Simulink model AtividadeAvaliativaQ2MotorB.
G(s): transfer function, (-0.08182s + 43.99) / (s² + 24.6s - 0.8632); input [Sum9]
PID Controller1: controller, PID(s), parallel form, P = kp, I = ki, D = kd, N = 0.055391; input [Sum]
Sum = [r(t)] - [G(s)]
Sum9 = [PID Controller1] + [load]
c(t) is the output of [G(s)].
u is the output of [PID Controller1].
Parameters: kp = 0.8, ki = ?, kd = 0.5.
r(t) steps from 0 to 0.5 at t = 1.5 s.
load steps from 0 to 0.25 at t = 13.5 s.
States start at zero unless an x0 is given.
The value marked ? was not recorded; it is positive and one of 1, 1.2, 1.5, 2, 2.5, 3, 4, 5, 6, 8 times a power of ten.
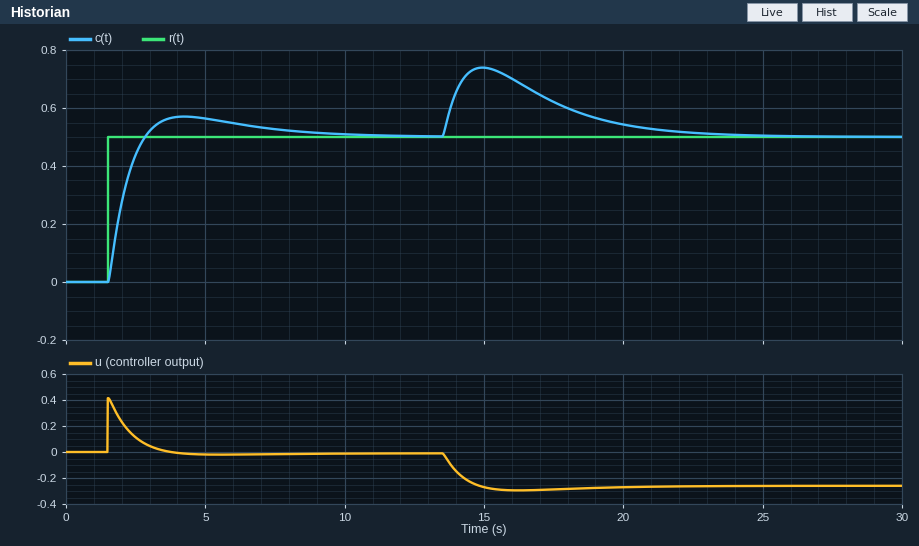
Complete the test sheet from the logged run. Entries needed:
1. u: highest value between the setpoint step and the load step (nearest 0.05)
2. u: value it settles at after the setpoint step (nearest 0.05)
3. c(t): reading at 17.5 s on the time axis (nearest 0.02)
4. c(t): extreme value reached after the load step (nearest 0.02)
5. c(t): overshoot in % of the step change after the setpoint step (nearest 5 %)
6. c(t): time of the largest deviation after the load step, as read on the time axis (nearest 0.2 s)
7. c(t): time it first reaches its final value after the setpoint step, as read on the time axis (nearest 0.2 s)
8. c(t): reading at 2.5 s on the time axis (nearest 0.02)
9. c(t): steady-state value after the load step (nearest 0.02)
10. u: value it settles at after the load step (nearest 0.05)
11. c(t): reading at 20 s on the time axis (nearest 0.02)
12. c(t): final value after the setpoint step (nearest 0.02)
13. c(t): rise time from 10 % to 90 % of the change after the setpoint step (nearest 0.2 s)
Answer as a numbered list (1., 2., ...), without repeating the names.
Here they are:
1. 0.40
2. 0.00
3. 0.62
4. 0.74
5. 15 %
6. 15.0 s
7. 2.8 s
8. 0.44
9. 0.50
10. -0.25
11. 0.54
12. 0.50
13. 1.0 s
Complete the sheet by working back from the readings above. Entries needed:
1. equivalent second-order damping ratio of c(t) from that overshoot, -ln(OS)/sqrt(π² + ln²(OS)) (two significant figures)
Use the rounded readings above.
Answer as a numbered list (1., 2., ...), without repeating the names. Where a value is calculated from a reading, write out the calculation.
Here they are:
1. ln(0.15) = -1.897; 1.897 / sqrt(9.870 + 3.599) = 0.52
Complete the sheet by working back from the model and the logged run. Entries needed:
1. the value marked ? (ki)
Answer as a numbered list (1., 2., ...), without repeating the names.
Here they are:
1. 0.25
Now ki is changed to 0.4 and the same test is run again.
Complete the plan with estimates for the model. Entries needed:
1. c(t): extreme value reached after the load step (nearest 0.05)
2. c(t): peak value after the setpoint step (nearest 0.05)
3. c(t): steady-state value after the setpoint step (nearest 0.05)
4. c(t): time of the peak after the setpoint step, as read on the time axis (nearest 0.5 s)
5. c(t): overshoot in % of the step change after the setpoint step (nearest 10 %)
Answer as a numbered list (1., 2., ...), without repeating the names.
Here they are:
1. 0.70
2. 0.60
3. 0.50
4. 4.0 s
5. 20 %
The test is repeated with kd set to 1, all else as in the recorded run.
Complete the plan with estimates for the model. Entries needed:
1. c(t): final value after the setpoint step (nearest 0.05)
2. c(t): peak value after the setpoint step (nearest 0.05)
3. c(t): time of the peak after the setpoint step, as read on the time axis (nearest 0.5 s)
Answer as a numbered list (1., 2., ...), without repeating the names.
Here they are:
1. 0.50
2. 0.55
3. 4.0 s
